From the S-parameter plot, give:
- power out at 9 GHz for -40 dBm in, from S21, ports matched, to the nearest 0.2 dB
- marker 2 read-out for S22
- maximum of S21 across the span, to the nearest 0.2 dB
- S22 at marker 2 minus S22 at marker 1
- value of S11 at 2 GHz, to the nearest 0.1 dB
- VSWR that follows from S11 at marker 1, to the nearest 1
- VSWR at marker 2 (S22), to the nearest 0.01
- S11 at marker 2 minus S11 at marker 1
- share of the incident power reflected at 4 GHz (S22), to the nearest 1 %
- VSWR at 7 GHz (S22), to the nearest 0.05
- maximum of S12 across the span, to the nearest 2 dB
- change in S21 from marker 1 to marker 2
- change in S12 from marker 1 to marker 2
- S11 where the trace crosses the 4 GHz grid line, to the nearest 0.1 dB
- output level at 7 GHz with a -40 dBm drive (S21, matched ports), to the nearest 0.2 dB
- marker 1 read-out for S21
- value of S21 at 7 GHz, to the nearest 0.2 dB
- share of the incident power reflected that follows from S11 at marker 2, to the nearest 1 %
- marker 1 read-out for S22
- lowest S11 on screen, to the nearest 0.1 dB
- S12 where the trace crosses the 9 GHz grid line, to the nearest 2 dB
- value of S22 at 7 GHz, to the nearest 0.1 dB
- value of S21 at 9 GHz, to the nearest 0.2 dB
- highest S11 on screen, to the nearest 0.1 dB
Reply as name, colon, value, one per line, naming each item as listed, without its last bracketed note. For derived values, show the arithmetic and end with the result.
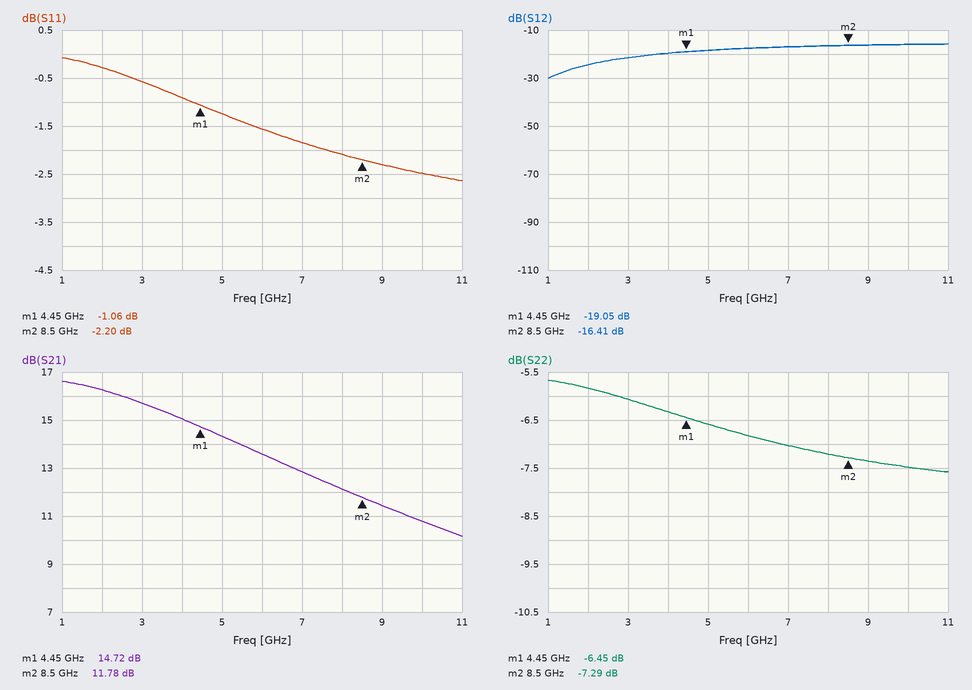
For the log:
power out at 9 GHz for -40 dBm in, from S21, ports matched, to the nearest 0.2 dB: -40 dBm + (11.4 dB) = -28.6 dBm
marker 2 read-out for S22: -7.29 dB
maximum of S21 across the span, to the nearest 0.2 dB: 16.6 dB
S22 at marker 2 minus S22 at marker 1: -7.29 − (-6.45) = -0.84 dB
value of S11 at 2 GHz, to the nearest 0.1 dB: -0.3 dB
VSWR that follows from S11 at marker 1, to the nearest 1: (1 + 0.8851)/(1 − 0.8851) ≈ 16
VSWR at marker 2 (S22), to the nearest 0.01: (1 + 0.4320)/(1 − 0.4320) ≈ 2.52
S11 at marker 2 minus S11 at marker 1: -2.2 − (-1.06) = -1.14 dB
share of the incident power reflected at 4 GHz (S22), to the nearest 1 %: 10^(-6.3/10) ≈ 23 %
VSWR at 7 GHz (S22), to the nearest 0.05: |Γ| = 10^(-7/20) = 0.4467; VSWR = (1 + 0.4467)/(1 − 0.4467) ≈ 2.61, so 2.60 to the nearest 0.05
maximum of S12 across the span, to the nearest 2 dB: -16 dB
change in S21 from marker 1 to marker 2: 11.78 − (14.72) = -2.94 dB
change in S12 from marker 1 to marker 2: -16.41 − (-19.05) = 2.64 dB
S11 where the trace crosses the 4 GHz grid line, to the nearest 0.1 dB: -0.9 dB
output level at 7 GHz with a -40 dBm drive (S21, matched ports), to the nearest 0.2 dB: -40 dBm + (12.8 dB) = -27.2 dBm
marker 1 read-out for S21: 14.72 dB
value of S21 at 7 GHz, to the nearest 0.2 dB: 12.8 dB
share of the incident power reflected that follows from S11 at marker 2, to the nearest 1 %: 10^(-2.2/10) ≈ 60 %
marker 1 read-out for S22: -6.45 dB
lowest S11 on screen, to the nearest 0.1 dB: -2.6 dB
S12 where the trace crosses the 9 GHz grid line, to the nearest 2 dB: -16 dB
value of S22 at 7 GHz, to the nearest 0.1 dB: -7.0 dB
value of S21 at 9 GHz, to the nearest 0.2 dB: 11.4 dB
highest S11 on screen, to the nearest 0.1 dB: -0.1 dB
